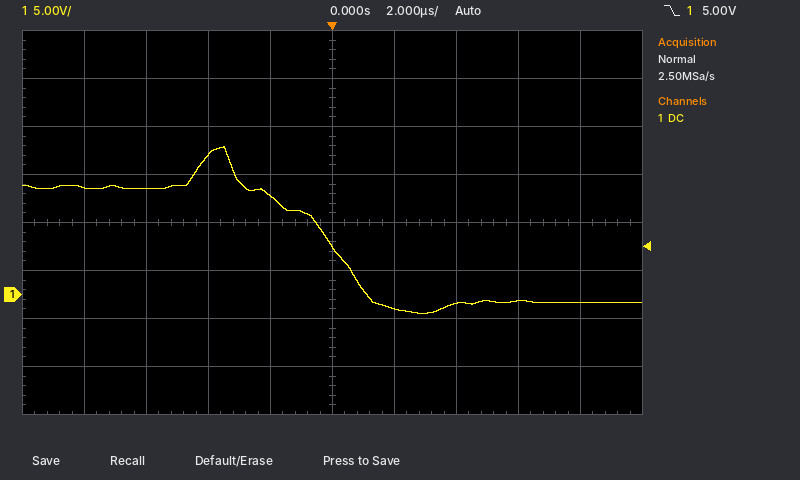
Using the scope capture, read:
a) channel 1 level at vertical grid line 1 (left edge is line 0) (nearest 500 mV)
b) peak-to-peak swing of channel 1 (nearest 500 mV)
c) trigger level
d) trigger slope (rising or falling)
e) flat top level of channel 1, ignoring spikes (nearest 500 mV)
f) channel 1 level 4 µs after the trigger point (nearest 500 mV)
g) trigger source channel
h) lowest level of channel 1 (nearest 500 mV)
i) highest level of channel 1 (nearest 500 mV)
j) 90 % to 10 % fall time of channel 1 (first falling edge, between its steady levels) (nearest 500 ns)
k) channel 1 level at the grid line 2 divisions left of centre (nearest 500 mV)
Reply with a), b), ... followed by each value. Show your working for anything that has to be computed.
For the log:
a) 11.0 V
b) 15.5 V − (-2.0 V) = 17.5 V
c) 5.00 V
d) falling
e) 11.0 V
f) -1.0 V
g) channel 1
h) -2.0 V
i) 15.5 V
j) 3.0 µs
k) 14.5 V
